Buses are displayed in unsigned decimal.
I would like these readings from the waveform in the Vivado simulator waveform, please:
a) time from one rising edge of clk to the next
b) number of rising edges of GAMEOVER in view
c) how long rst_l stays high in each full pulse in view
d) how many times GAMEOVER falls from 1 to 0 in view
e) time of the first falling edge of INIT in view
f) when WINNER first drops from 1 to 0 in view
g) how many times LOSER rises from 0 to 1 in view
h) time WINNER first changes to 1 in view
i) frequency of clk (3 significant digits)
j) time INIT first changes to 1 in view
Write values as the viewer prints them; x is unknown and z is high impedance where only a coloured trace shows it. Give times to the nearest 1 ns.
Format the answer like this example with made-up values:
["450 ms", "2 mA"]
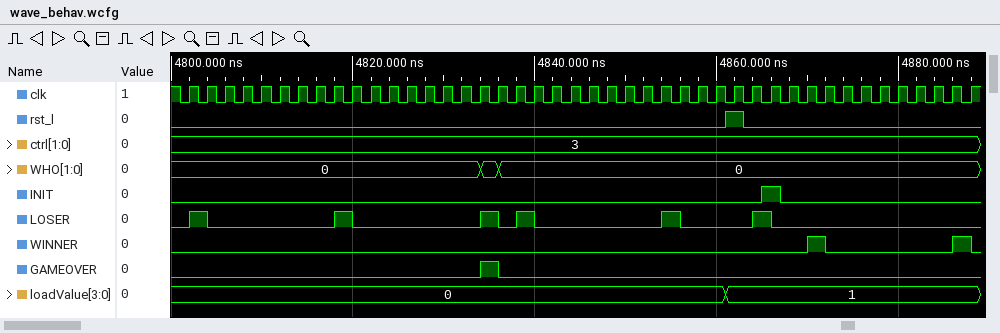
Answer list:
["2 ns", "1", "2 ns", "1", "4867 ns", "4872 ns", "6", "4870 ns", "500 MHz", "4865 ns"]
